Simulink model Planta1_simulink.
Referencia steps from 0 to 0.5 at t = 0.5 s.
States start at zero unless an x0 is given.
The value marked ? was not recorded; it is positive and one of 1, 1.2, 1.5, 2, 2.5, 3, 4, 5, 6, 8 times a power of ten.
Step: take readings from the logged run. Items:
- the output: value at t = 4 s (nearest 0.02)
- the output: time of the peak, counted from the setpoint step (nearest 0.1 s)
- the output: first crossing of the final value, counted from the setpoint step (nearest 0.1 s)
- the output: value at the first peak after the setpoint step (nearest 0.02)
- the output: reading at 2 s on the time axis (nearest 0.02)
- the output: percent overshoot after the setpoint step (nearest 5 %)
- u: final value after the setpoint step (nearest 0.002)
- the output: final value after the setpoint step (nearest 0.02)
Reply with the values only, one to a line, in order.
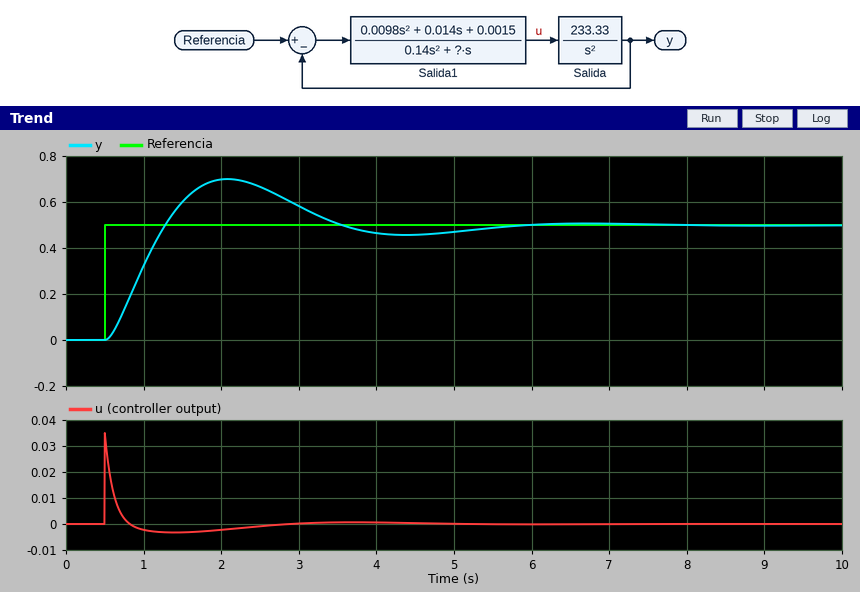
0.46
1.6 s
0.8 s
0.70
0.70
40 %
0.000
0.50
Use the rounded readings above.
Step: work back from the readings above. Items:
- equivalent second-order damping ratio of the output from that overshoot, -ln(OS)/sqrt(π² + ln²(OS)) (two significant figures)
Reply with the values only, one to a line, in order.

0.28
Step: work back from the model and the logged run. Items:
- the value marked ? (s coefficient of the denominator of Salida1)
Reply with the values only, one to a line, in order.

1.5
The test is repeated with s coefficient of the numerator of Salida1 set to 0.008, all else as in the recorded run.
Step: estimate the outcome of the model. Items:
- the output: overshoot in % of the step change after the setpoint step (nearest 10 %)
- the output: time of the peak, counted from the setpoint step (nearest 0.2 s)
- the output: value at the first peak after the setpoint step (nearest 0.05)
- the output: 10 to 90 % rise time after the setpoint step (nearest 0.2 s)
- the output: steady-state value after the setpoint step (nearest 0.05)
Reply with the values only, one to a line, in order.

30 %
2.0 s
0.65
0.6 s
0.50
